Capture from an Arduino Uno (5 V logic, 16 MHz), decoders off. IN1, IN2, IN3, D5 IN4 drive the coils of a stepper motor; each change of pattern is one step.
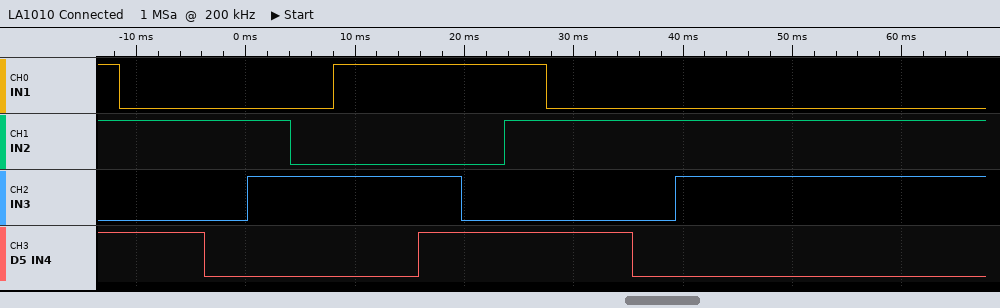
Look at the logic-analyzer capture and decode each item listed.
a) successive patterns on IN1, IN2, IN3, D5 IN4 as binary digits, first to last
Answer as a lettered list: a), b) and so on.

a) 1101 0101 0100 0110 0010 1010 1011 1001 1101 0101 0100 0110
